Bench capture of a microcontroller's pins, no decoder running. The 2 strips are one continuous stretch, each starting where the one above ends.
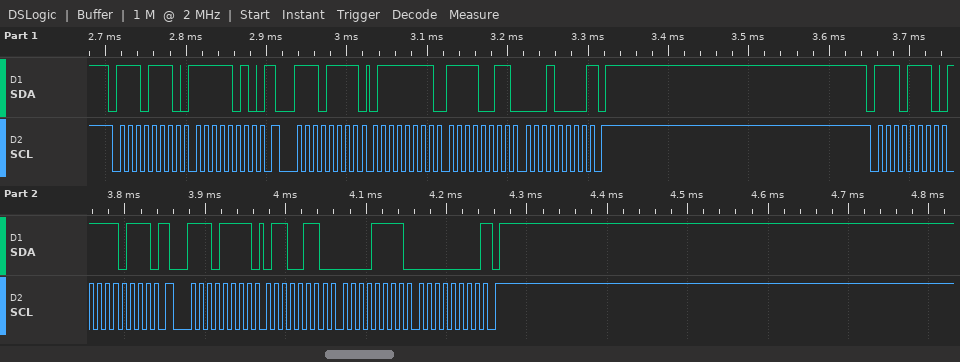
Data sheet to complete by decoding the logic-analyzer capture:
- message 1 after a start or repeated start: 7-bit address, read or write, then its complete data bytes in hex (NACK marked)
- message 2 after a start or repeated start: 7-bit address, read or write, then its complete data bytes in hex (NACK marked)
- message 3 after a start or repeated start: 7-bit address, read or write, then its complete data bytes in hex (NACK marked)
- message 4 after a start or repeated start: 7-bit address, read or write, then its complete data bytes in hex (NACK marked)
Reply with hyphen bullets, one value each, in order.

- 0x77 write: FA
- 0x77 read: 7F F3 10 NACK
- 0x77 write: F7
- 0x77 read: 66 0F 00 NACK
